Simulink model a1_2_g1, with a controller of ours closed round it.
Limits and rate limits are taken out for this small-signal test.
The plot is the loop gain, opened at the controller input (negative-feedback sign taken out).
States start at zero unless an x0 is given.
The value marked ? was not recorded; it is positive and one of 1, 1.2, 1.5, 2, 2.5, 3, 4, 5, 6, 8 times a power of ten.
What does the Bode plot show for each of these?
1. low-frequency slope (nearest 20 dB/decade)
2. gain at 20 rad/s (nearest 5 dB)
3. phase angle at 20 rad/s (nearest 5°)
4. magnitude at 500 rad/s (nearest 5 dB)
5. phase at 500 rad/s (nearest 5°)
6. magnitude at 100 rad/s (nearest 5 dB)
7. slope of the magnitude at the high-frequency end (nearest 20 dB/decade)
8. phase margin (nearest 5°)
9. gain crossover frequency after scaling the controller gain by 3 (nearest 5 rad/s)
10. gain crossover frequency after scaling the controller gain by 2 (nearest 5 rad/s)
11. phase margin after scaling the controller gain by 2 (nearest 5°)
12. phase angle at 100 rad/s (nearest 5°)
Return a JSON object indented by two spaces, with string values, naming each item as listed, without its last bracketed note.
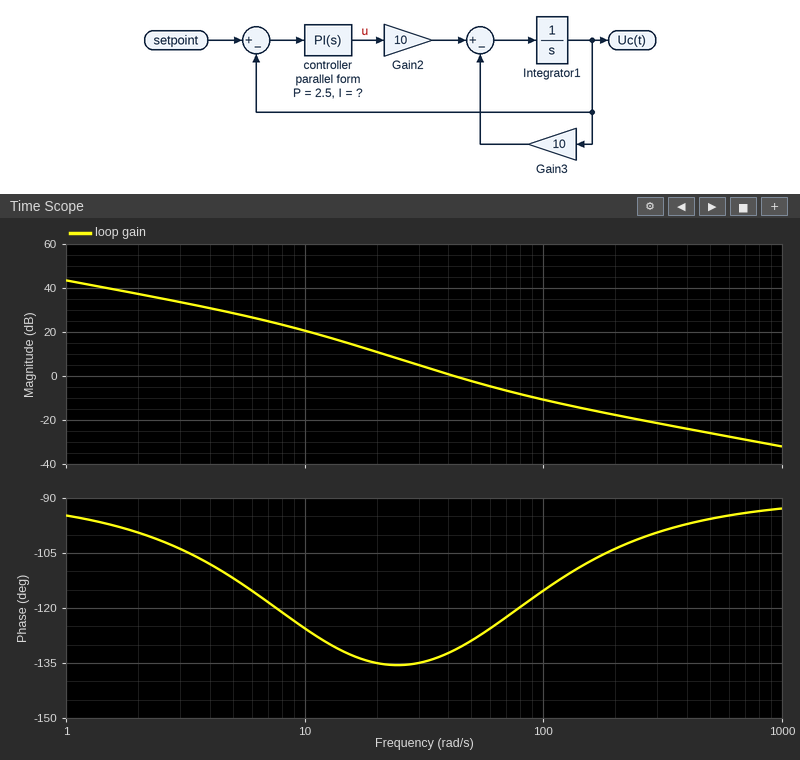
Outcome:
{
  "low-frequency slope": "-20 dB/decade",
  "gain at 20 rad/s": "10 dB",
  "phase angle at 20 rad/s": "-135°",
  "magnitude at 500 rad/s": "-25 dB",
  "phase at 500 rad/s": "-95°",
  "magnitude at 100 rad/s": "-10 dB",
  "slope of the magnitude at the high-frequency end": "-20 dB/decade",
  "phase margin": "50°",
  "gain crossover frequency after scaling the controller gain by 3": "90 rad/s",
  "gain crossover frequency after scaling the controller gain by 2": "65 rad/s",
  "phase margin after scaling the controller gain by 2": "55°",
  "phase angle at 100 rad/s": "-115°"
}
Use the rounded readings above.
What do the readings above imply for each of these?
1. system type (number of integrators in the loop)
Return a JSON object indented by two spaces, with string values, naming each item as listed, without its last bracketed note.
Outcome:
{
  "system type": "1"
}
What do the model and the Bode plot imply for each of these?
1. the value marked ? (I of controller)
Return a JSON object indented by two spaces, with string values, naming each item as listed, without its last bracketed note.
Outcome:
{
  "the value marked ?": "150"
}
